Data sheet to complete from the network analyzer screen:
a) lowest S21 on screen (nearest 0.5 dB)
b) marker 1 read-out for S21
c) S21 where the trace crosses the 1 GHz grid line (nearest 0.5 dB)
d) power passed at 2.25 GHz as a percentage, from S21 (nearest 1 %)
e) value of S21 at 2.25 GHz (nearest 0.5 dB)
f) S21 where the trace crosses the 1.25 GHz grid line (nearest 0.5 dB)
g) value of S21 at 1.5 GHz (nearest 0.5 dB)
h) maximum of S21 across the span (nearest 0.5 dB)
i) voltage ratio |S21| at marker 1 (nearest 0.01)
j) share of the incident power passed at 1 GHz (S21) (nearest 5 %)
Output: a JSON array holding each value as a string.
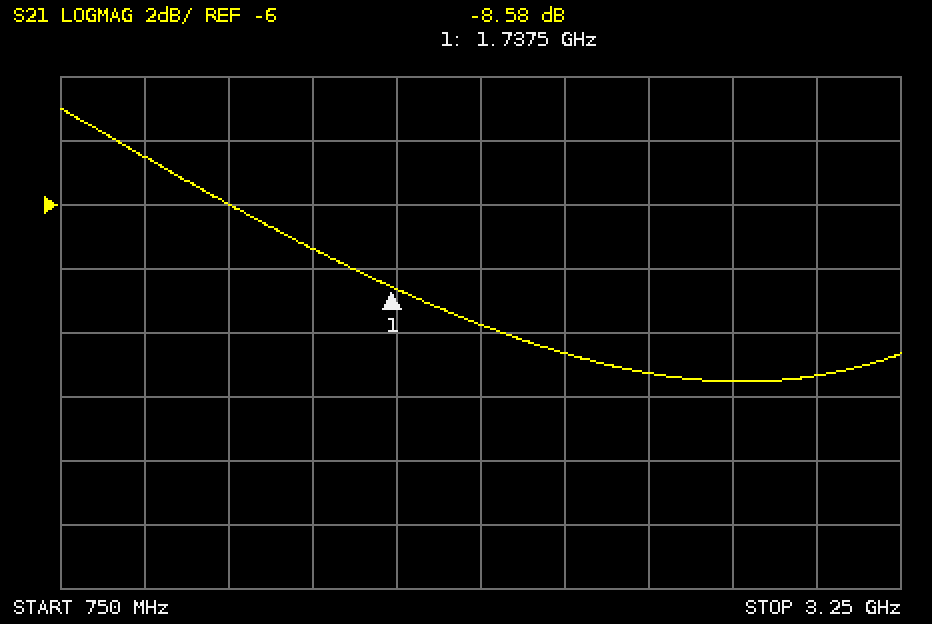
["-11.5 dB", "-8.58 dB", "-4.5 dB", "9 %", "-10.5 dB", "-6.0 dB", "-7.5 dB", "-3.0 dB", "0.37", "35 %"]
